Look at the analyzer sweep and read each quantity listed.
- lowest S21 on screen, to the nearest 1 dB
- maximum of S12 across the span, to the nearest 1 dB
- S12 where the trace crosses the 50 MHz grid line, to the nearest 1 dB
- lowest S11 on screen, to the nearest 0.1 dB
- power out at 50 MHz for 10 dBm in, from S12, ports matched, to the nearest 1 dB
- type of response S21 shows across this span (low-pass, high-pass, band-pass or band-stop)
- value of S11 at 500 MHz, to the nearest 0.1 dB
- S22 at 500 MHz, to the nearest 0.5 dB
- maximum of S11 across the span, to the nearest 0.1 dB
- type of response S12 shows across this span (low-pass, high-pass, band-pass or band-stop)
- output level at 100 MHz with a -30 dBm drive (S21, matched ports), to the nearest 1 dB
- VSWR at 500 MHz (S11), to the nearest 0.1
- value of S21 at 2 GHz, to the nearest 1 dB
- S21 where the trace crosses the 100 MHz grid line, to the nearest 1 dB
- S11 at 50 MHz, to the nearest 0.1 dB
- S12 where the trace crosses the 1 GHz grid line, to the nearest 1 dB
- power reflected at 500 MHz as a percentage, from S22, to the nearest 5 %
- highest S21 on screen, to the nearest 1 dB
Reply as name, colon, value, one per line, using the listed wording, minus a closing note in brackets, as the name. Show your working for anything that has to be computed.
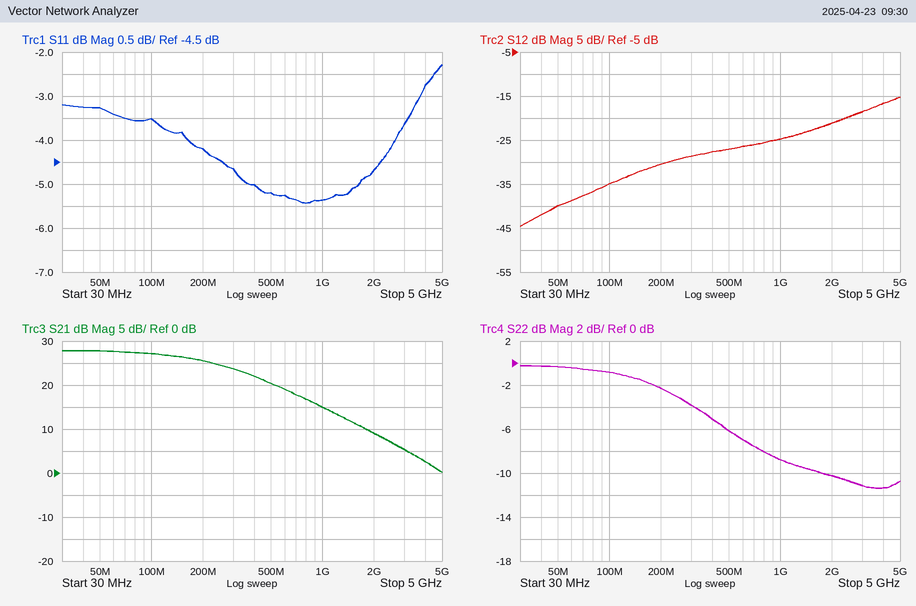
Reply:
lowest S21 on screen, to the nearest 1 dB: 0 dB
maximum of S12 across the span, to the nearest 1 dB: -15 dB
S12 where the trace crosses the 50 MHz grid line, to the nearest 1 dB: -40 dB
lowest S11 on screen, to the nearest 0.1 dB: -5.4 dB
power out at 50 MHz for 10 dBm in, from S12, ports matched, to the nearest 1 dB: 10 dBm + (-40 dB) = -30 dBm
type of response S21 shows across this span: low-pass
value of S11 at 500 MHz, to the nearest 0.1 dB: -5.2 dB
S22 at 500 MHz, to the nearest 0.5 dB: -6.0 dB
maximum of S11 across the span, to the nearest 0.1 dB: -2.3 dB
type of response S12 shows across this span: high-pass
output level at 100 MHz with a -30 dBm drive (S21, matched ports), to the nearest 1 dB: -30 dBm + (27 dB) = -3 dBm
VSWR at 500 MHz (S11), to the nearest 0.1: |Γ| = 10^(-5.2/20) = 0.5495; VSWR = (1 + 0.5495)/(1 − 0.5495) ≈ 3.4
value of S21 at 2 GHz, to the nearest 1 dB: 9 dB
S21 where the trace crosses the 100 MHz grid line, to the nearest 1 dB: 27 dB
S11 at 50 MHz, to the nearest 0.1 dB: -3.3 dB
S12 where the trace crosses the 1 GHz grid line, to the nearest 1 dB: -25 dB
power reflected at 500 MHz as a percentage, from S22, to the nearest 5 %: 10^(-6/10) ≈ 25 %
highest S21 on screen, to the nearest 1 dB: 28 dB
